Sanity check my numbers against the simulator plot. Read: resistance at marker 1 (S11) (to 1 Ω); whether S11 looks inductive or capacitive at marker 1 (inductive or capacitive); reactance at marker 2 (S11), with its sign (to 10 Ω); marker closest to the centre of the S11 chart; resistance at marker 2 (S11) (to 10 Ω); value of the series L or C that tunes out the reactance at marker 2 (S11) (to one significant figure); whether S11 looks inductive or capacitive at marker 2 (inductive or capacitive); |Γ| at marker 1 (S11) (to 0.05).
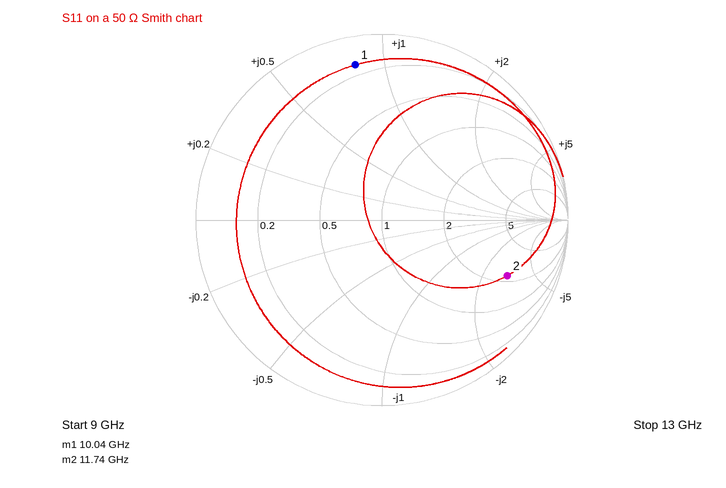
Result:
7 Ω
inductive
-150 Ω
marker 2
120 Ω
2 nH
capacitive
0.85
